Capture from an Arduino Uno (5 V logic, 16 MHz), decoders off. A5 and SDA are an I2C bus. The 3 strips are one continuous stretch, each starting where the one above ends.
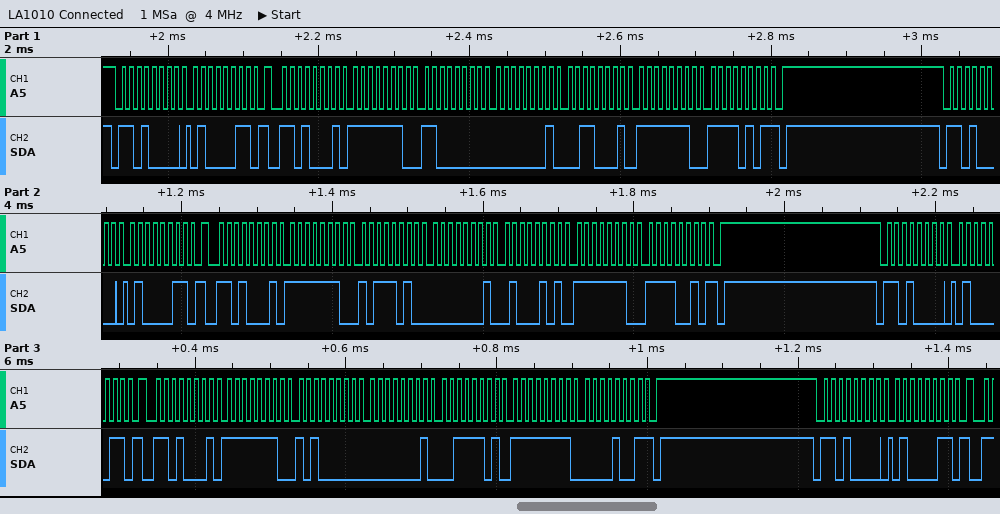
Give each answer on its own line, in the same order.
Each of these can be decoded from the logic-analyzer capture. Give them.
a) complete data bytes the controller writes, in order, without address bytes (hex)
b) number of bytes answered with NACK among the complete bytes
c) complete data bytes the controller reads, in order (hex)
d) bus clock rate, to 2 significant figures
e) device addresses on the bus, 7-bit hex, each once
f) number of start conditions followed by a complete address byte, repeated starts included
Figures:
43 43 43 43
3
FE C0 01 31 FE F5 FE BA 01 45 FE F2 FE A0 01 3D FF 09
100 kHz
0x68
7
